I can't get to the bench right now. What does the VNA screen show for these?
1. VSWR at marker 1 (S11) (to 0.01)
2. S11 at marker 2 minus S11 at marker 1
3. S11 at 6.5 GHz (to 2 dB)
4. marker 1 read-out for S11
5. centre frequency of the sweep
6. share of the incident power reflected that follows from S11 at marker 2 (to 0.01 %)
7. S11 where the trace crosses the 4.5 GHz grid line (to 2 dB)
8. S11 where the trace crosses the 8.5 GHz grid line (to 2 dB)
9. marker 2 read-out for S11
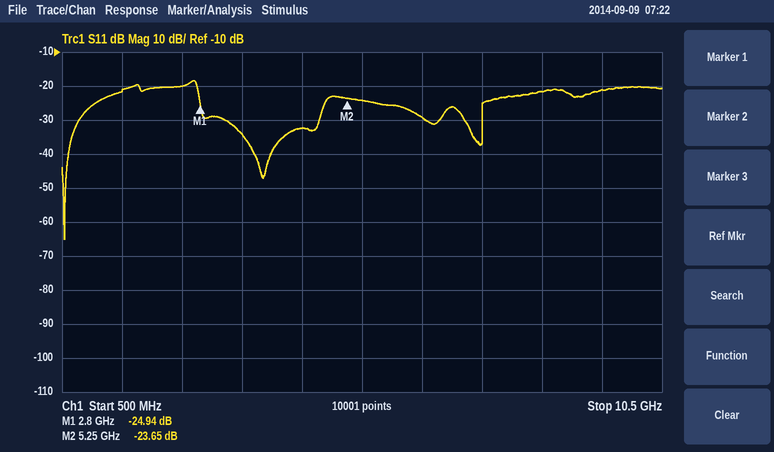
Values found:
1.12
1.29 dB
-30 dB
-24.94 dB
5.5 GHz
0.43 %
-32 dB
-22 dB
-23.65 dB
